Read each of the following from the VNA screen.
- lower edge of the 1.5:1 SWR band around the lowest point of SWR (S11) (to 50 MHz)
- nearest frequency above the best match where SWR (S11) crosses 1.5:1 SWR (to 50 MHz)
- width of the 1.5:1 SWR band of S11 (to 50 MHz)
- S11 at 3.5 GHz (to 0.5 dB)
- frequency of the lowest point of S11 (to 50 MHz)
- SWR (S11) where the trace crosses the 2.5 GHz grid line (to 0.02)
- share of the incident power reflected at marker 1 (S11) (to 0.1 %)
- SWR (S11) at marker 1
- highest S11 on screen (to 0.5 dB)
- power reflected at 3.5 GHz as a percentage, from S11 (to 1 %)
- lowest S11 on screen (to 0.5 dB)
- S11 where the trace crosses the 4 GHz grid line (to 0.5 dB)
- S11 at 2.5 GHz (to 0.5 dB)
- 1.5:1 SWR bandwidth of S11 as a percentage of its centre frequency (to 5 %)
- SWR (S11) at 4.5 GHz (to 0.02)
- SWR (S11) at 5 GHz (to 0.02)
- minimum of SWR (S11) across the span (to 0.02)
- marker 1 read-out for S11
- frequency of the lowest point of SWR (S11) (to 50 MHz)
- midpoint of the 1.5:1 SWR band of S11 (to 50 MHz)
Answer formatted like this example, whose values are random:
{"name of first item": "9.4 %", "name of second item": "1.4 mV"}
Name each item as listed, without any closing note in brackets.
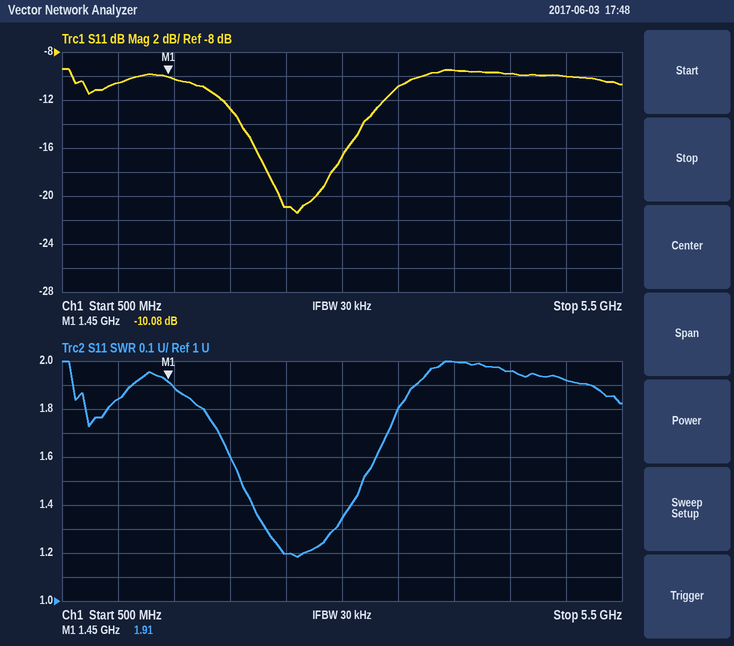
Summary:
{"lower edge of the 1.5:1 SWR band around the lowest point of SWR (S11)": "2.10 GHz", "nearest frequency above the best match where SWR (S11) crosses 1.5:1 SWR": "3.20 GHz", "width of the 1.5:1 SWR band of S11": "1.10 GHz", "S11 at 3.5 GHz": "-11.0 dB", "frequency of the lowest point of S11": "2.60 GHz", "SWR (S11) where the trace crosses the 2.5 GHz grid line": "1.20", "share of the incident power reflected at marker 1 (S11)": "9.8 %", "SWR (S11) at marker 1": "1.91", "highest S11 on screen": "-9.5 dB", "power reflected at 3.5 GHz as a percentage, from S11": "8 %", "lowest S11 on screen": "-21.5 dB", "S11 where the trace crosses the 4 GHz grid line": "-9.5 dB", "S11 at 2.5 GHz": "-21.0 dB", "1.5:1 SWR bandwidth of S11 as a percentage of its centre frequency": "40 %", "SWR (S11) at 4.5 GHz": "1.96", "SWR (S11) at 5 GHz": "1.92", "minimum of SWR (S11) across the span": "1.18", "marker 1 read-out for S11": "-10.08 dB", "frequency of the lowest point of SWR (S11)": "2.60 GHz", "midpoint of the 1.5:1 SWR band of S11": "2.65 GHz"}
